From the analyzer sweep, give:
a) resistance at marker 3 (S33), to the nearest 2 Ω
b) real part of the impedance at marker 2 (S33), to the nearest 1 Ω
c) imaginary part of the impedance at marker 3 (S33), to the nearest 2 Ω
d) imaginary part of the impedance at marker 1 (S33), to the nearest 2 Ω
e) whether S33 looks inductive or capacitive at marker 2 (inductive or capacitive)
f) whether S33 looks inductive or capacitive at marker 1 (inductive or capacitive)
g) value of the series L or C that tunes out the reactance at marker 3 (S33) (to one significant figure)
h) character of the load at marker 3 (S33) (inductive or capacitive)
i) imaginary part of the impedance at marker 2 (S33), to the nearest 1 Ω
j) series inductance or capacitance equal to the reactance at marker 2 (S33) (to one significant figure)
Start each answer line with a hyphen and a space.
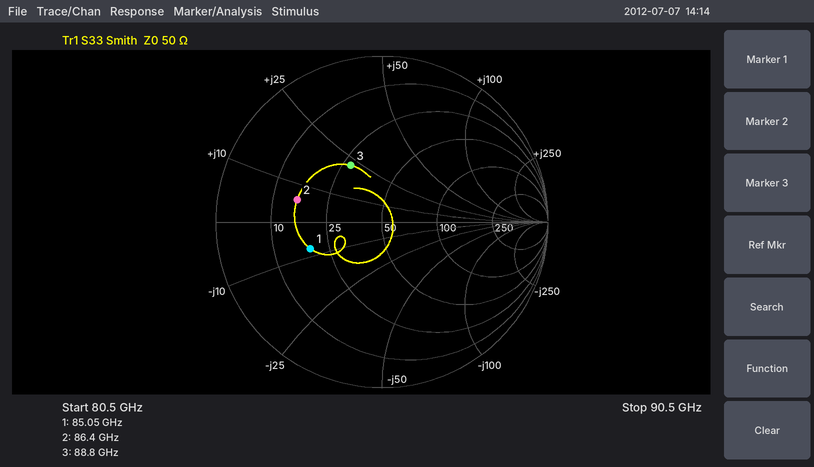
- 28 Ω
- 16 Ω
- +22 Ω
- -8 Ω
- inductive
- capacitive
- 80 fF
- inductive
- +6 Ω
- 10 pH
